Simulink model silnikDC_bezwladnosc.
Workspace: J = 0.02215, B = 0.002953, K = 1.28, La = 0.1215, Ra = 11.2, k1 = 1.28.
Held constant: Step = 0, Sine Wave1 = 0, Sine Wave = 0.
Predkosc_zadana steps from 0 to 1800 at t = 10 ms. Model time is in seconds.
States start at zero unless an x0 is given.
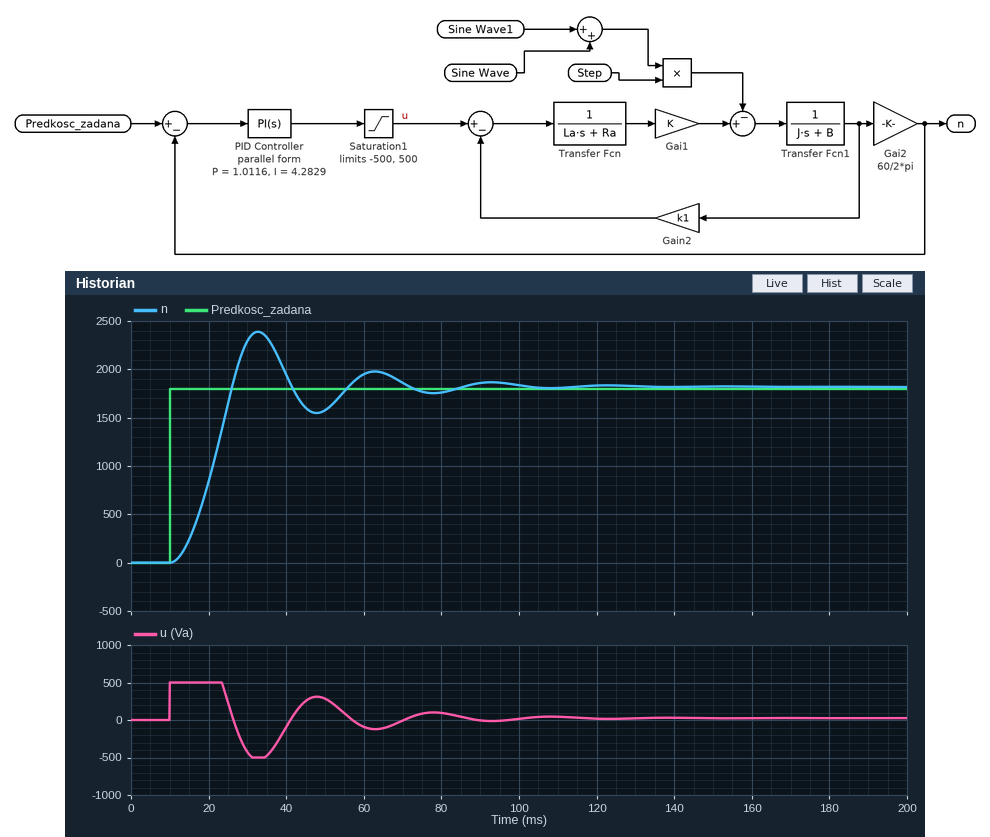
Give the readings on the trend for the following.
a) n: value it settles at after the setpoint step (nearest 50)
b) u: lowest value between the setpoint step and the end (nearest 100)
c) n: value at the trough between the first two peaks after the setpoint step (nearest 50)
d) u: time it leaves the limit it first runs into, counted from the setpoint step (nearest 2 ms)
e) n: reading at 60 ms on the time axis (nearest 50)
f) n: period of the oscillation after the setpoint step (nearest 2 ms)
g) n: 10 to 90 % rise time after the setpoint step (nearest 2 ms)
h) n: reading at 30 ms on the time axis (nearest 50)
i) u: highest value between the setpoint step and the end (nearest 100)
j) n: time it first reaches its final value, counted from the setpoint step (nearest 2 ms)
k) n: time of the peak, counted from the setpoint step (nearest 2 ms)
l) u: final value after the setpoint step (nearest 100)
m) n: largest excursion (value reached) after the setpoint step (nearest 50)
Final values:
1800
-500
1550
14 ms
1950
30 ms
10 ms
2300
500
16 ms
22 ms
0
2400
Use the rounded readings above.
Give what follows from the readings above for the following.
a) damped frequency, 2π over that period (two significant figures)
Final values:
0.21 rad/ms
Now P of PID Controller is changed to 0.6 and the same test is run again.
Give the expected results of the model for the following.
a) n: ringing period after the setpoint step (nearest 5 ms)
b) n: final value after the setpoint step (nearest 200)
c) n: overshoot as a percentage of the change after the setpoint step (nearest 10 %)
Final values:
40 ms
1800
40 %
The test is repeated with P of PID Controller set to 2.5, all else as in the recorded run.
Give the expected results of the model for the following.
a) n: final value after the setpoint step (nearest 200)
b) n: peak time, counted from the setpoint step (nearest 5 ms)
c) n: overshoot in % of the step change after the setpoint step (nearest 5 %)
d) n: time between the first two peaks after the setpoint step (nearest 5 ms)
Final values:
1800
20 ms
30 %
20 ms
